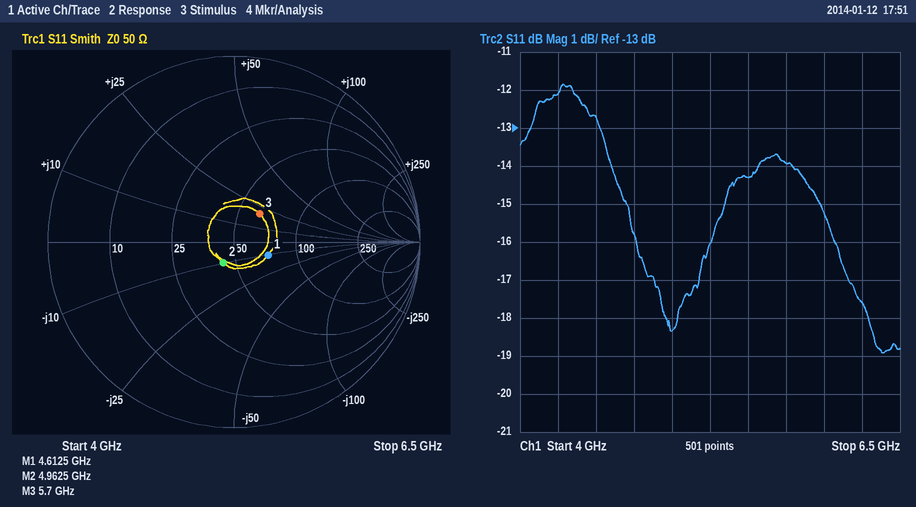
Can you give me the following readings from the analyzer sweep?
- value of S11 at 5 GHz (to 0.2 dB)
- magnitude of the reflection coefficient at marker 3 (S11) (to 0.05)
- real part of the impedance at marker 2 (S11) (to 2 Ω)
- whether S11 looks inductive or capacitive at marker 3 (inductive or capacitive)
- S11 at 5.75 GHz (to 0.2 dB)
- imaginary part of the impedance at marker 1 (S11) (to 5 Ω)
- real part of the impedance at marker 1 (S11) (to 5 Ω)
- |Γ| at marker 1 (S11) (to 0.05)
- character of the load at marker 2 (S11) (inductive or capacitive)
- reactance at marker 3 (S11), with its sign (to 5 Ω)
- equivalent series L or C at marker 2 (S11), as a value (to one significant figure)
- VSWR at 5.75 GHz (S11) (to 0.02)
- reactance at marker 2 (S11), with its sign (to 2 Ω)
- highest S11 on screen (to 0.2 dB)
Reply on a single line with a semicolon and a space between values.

-18.4 dB; 0.20; 44 Ω; inductive; -14.0 dB; -10 Ω; 70 Ω; 0.20; capacitive; +20 Ω; 3 pF; 1.50; -10 Ω; -11.8 dB
